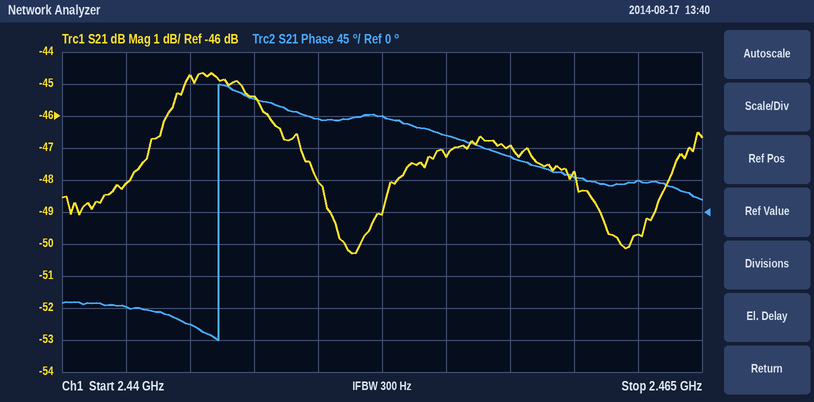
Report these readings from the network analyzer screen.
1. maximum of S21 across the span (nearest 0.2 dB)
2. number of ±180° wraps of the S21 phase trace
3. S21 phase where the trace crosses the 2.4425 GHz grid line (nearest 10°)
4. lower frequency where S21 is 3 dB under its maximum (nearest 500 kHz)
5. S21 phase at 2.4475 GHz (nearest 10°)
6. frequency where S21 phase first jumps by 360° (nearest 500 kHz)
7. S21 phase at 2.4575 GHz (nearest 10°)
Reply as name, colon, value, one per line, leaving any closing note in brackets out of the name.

maximum of S21 across the span: -44.6 dB
number of ±180° wraps of the S21 phase trace: 1
S21 phase where the trace crosses the 2.4425 GHz grid line: -130°
lower frequency where S21 is 3 dB under its maximum: 2.4430 GHz
S21 phase at 2.4475 GHz: 160°
frequency where S21 phase first jumps by 360°: 2.4460 GHz
S21 phase at 2.4575 GHz: 80°
